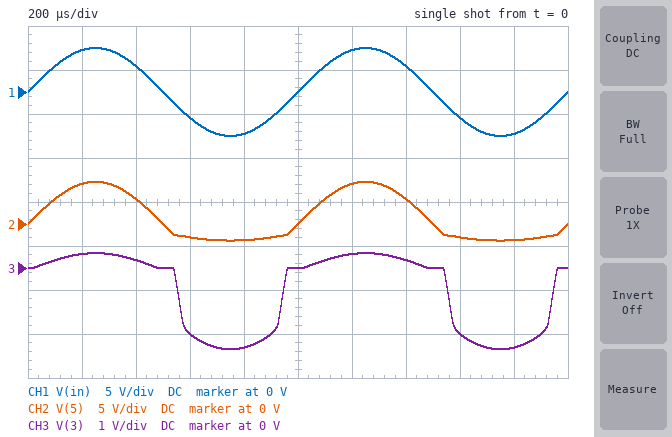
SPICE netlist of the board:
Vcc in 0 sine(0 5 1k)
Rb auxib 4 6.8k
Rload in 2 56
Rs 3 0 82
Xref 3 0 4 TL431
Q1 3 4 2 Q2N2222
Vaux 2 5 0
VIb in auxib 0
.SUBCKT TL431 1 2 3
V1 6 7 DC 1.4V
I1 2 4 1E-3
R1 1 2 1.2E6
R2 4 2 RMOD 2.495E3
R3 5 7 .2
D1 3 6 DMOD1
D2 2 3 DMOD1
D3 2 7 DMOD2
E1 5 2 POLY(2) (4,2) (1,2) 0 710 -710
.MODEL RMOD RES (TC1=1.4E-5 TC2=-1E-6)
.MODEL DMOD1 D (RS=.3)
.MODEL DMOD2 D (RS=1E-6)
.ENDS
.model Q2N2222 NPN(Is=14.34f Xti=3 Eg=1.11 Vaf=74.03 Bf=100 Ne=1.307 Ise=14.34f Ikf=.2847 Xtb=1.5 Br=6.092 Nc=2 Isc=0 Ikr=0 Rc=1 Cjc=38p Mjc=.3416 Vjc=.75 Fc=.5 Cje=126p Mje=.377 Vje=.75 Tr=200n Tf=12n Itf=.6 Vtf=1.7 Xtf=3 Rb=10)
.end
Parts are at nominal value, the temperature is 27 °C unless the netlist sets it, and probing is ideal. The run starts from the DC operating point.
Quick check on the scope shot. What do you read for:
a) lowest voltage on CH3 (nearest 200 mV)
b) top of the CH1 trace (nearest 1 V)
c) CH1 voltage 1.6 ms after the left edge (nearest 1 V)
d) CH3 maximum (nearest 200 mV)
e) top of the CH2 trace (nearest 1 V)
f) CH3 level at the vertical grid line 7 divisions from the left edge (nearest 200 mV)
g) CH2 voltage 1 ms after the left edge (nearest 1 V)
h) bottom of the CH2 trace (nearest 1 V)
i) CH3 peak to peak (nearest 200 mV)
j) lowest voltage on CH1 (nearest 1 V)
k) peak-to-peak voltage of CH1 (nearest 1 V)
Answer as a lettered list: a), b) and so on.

a) -1.8 V
b) 5 V
c) -3 V
d) 400 mV
e) 5 V
f) 200 mV
g) 0 V
h) -2 V
i) 2.2 V
j) -5 V
k) 10 V
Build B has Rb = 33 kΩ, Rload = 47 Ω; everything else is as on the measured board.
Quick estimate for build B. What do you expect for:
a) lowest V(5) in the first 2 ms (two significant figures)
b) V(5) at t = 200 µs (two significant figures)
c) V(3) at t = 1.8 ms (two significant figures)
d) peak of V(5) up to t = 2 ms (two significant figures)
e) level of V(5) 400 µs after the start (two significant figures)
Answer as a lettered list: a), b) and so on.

a) -2.0 V
b) 4.7 V
c) -1.9 V
d) 5.0 V
e) 2.9 V
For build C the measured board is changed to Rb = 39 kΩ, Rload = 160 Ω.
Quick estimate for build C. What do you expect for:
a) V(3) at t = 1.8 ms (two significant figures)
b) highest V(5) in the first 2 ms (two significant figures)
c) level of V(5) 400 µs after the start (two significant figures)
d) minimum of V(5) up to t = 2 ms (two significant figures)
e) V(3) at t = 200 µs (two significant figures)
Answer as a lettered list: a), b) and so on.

a) -1.4 V
b) 4.9 V
c) 2.9 V
d) -1.5 V
e) 60 mV
